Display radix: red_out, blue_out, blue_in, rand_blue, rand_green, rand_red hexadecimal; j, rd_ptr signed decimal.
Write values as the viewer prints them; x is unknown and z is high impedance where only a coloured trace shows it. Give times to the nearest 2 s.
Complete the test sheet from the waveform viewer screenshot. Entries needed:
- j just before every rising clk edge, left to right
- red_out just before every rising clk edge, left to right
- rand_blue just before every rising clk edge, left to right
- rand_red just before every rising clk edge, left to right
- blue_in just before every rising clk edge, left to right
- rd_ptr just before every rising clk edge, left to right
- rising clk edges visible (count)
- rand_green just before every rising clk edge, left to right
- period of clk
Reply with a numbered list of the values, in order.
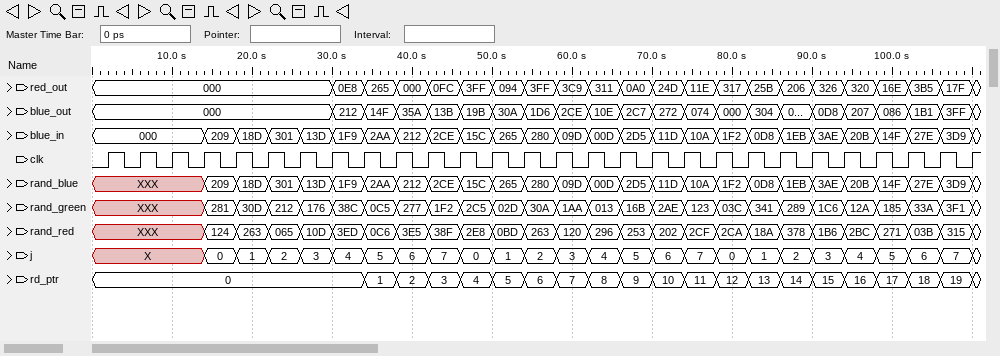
1. X, X, X, X, 0, 1, 2, 3, 4, 5, 6, 7, 0, 1, 2, 3, 4, 5, 6, 7, 0, 1, 2, 3, 4, 5, 6, 7
2. 000, 000, 000, 000, 000, 000, 000, 000, 0E8, 265, 000, 0FC, 3FF, 094, 3FF, 3C9, 311, 0A0, 24D, 11E, 317, 25B, 206, 326, 320, 16E, 3B5, 17F
3. XXX, XXX, XXX, XXX, 209, 18D, 301, 13D, 1F9, 2AA, 212, 2CE, 15C, 265, 280, 09D, 00D, 2D5, 11D, 10A, 1F2, 0D8, 1EB, 3AE, 20B, 14F, 27E, 3D9
4. XXX, XXX, XXX, XXX, 124, 263, 065, 10D, 3ED, 0C6, 3E5, 38F, 2E8, 0BD, 263, 120, 296, 253, 202, 2CF, 2CA, 18A, 378, 1B6, 2BC, 271, 03B, 315
5. 000, 000, 000, 000, 209, 18D, 301, 13D, 1F9, 2AA, 212, 2CE, 15C, 265, 280, 09D, 00D, 2D5, 11D, 10A, 1F2, 0D8, 1EB, 3AE, 20B, 14F, 27E, 3D9
6. 0, 0, 0, 0, 0, 0, 0, 0, 0, 1, 2, 3, 4, 5, 6, 7, 8, 9, 10, 11, 12, 13, 14, 15, 16, 17, 18, 19
7. 28
8. XXX, XXX, XXX, XXX, 281, 30D, 212, 176, 38C, 0C5, 277, 1F2, 2C5, 02D, 30A, 1AA, 013, 16B, 2AE, 123, 03C, 341, 289, 1C6, 12A, 185, 33A, 3F1
9. 4 s
